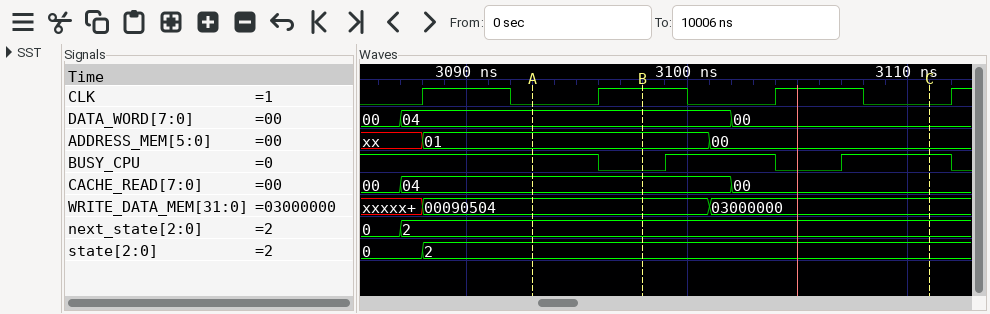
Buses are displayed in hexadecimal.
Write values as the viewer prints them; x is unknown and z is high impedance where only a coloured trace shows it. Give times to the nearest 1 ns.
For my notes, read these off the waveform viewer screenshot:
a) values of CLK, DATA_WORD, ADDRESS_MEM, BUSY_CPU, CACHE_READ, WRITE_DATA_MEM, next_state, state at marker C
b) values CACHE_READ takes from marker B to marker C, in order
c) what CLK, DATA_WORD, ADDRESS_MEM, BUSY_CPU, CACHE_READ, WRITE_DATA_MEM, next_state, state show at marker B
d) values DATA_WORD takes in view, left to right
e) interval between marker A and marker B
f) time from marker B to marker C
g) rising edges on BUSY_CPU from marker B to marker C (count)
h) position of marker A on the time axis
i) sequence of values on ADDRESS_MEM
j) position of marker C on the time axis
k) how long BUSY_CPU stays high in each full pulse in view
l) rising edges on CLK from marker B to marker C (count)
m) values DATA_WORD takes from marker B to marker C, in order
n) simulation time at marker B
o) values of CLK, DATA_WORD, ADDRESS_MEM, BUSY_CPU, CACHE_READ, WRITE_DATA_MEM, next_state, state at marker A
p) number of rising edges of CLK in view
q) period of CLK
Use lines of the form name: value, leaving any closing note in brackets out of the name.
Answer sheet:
values of CLK, DATA_WORD, ADDRESS_MEM, BUSY_CPU, CACHE_READ, WRITE_DATA_MEM, next_state, state at marker C: CLK=0, DATA_WORD=00, ADDRESS_MEM=00, BUSY_CPU=1, CACHE_READ=00, WRITE_DATA_MEM=03000000, next_state=2, state=2
values CACHE_READ takes from marker B to marker C, in order: 04, 00
what CLK, DATA_WORD, ADDRESS_MEM, BUSY_CPU, CACHE_READ, WRITE_DATA_MEM, next_state, state show at marker B: CLK=1, DATA_WORD=04, ADDRESS_MEM=01, BUSY_CPU=0, CACHE_READ=04, WRITE_DATA_MEM=00090504, next_state=2, state=2
values DATA_WORD takes in view, left to right: 00, 04, 00
interval between marker A and marker B: 5 ns
time from marker B to marker C: 13 ns
rising edges on BUSY_CPU from marker B to marker C: 2
position of marker A on the time axis: 3093 ns
sequence of values on ADDRESS_MEM: xx, 01, 00
position of marker C on the time axis: 3111 ns
how long BUSY_CPU stays high in each full pulse in view: 5 ns, 5 ns
rising edges on CLK from marker B to marker C: 1
values DATA_WORD takes from marker B to marker C, in order: 04, 00
simulation time at marker B: 3098 ns
values of CLK, DATA_WORD, ADDRESS_MEM, BUSY_CPU, CACHE_READ, WRITE_DATA_MEM, next_state, state at marker A: CLK=0, DATA_WORD=04, ADDRESS_MEM=01, BUSY_CPU=1, CACHE_READ=04, WRITE_DATA_MEM=00090504, next_state=2, state=2
number of rising edges of CLK in view: 4
period of CLK: 8 ns
